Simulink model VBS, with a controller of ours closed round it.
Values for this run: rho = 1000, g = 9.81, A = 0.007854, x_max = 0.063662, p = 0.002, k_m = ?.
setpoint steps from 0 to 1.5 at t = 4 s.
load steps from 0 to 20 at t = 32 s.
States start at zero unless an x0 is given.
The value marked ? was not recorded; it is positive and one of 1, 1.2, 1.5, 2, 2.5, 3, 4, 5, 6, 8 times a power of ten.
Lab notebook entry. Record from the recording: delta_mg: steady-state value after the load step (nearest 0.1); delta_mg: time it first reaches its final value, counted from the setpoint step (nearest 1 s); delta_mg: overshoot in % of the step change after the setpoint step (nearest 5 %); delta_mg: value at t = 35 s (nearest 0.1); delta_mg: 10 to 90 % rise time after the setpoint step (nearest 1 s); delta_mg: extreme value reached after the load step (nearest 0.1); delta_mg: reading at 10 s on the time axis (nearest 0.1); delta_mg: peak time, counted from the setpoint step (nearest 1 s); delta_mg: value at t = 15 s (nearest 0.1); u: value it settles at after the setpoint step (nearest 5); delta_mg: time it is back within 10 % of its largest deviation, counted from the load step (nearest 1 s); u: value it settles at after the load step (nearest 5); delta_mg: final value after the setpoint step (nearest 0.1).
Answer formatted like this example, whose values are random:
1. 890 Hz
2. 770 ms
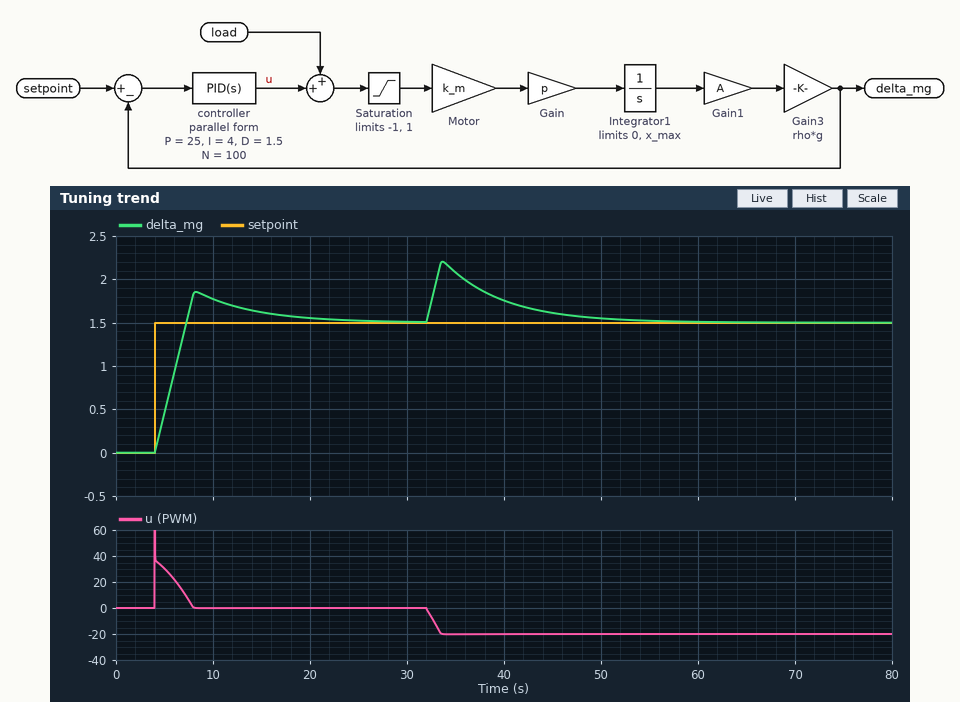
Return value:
1. 1.5
2. 3 s
3. 25 %
4. 2.1
5. 3 s
6. 2.2
7. 1.8
8. 4 s
9. 1.6
10. 0
11. 16 s
12. -20
13. 1.5
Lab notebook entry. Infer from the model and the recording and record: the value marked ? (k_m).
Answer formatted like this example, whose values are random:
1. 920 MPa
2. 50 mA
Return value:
1. 3
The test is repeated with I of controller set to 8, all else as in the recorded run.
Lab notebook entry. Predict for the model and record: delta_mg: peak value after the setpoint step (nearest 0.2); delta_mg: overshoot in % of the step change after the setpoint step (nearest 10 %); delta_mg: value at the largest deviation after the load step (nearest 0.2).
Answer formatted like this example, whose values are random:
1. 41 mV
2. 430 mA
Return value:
1. 2.2
2. 40 %
3. 2.2
